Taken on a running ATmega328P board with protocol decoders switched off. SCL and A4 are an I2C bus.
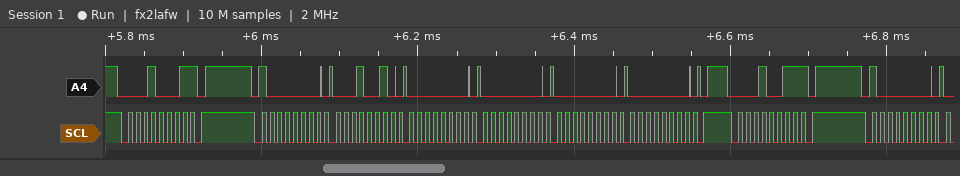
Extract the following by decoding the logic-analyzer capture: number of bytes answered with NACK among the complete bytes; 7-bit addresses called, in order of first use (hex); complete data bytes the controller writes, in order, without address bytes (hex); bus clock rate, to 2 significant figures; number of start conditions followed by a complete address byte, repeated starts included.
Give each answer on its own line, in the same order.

2
0x08 0x40 0x09
12 00 00 00 00
100 kHz
4
